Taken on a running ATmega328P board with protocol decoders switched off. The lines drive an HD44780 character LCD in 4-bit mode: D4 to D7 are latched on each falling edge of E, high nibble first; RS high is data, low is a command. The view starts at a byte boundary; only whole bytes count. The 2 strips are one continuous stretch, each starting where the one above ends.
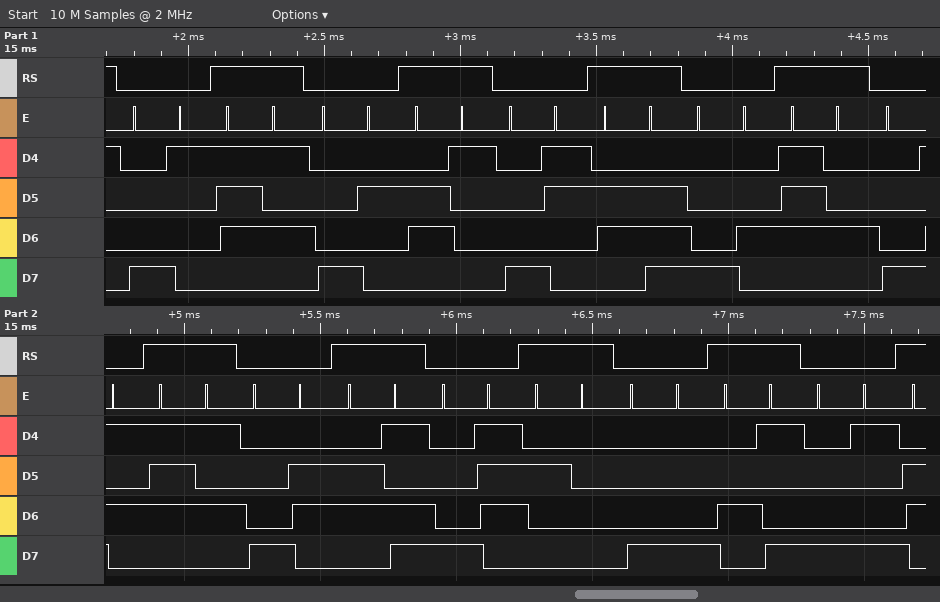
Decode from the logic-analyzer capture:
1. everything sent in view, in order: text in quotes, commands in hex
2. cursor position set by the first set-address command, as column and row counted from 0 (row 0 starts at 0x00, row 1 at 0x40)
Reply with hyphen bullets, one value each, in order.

- 0x81 "u" 0x82 "a" 0x83 "n" 0x84 "t" 0x85 "u" 0x86 "m" 0x87 " " 0x88 "I" 0x89
- column 1, row 0
